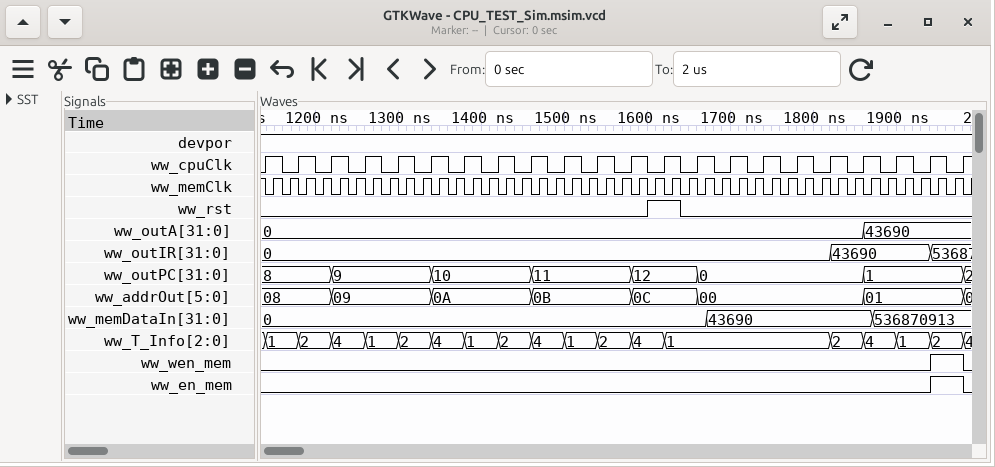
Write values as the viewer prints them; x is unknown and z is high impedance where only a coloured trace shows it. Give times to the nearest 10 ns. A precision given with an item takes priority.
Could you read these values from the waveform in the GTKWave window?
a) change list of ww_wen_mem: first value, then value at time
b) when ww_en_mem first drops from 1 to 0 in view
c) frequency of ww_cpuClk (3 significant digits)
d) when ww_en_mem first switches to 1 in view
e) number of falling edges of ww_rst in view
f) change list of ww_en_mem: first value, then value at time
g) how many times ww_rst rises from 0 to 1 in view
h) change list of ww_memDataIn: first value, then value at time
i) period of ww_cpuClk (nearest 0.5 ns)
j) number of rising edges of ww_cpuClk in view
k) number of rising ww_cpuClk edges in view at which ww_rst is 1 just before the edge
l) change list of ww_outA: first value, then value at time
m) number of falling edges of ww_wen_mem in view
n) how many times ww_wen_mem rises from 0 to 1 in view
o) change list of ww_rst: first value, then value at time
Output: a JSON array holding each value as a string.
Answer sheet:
["0, 1 at 1940 ns, 0 at 1980 ns", "1980 ns", "25.0 MHz", "1940 ns", "1", "0, 1 at 1940 ns, 0 at 1980 ns", "1", "0, 43690 at 1670 ns, 536870913 at 1870 ns", "40 ns", "22", "1", "0, 43690 at 1860 ns", "1", "1", "0, 1 at 1600 ns, 0 at 1640 ns"]
